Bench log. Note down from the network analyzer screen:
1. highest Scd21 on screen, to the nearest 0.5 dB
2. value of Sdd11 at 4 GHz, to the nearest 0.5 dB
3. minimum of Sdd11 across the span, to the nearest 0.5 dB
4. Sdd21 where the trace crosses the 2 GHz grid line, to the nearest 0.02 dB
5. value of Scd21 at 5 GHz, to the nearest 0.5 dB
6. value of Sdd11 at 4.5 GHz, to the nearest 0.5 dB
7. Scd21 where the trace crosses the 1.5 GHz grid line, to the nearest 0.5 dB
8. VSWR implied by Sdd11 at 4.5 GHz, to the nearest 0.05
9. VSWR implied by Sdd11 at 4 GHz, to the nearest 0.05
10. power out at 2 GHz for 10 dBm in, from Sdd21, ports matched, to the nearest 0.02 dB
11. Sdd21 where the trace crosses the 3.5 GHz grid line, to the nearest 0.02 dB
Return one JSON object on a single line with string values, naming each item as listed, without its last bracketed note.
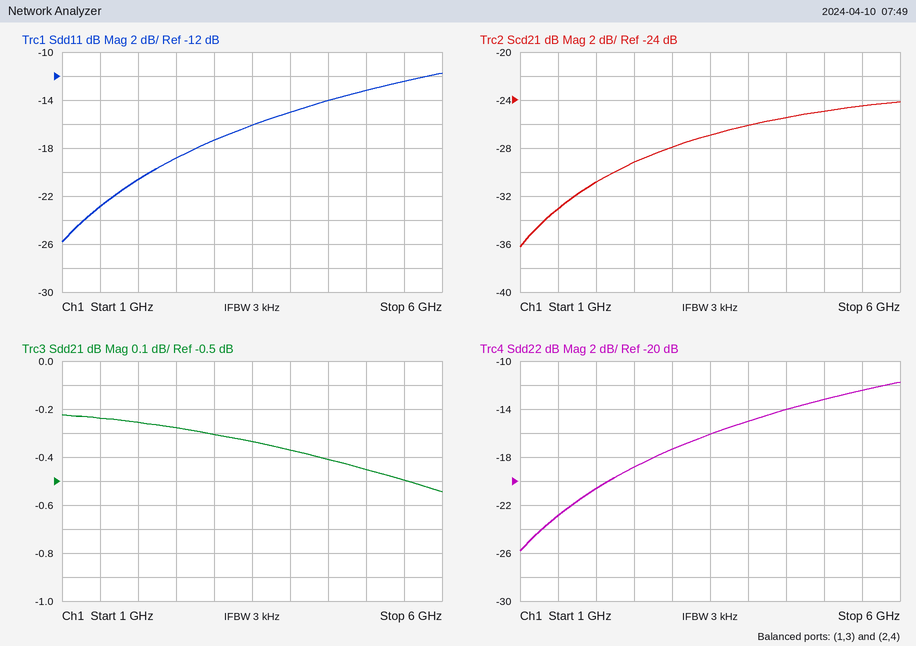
{"highest Scd21 on screen, to the nearest 0.5 dB": "-24.0 dB", "value of Sdd11 at 4 GHz, to the nearest 0.5 dB": "-15.0 dB", "minimum of Sdd11 across the span, to the nearest 0.5 dB": "-26.0 dB", "Sdd21 where the trace crosses the 2 GHz grid line, to the nearest 0.02 dB": "-0.26 dB", "value of Scd21 at 5 GHz, to the nearest 0.5 dB": "-25.0 dB", "value of Sdd11 at 4.5 GHz, to the nearest 0.5 dB": "-14.0 dB", "Scd21 where the trace crosses the 1.5 GHz grid line, to the nearest 0.5 dB": "-33.0 dB", "VSWR implied by Sdd11 at 4.5 GHz, to the nearest 0.05": "1.50", "VSWR implied by Sdd11 at 4 GHz, to the nearest 0.05": "1.45", "power out at 2 GHz for 10 dBm in, from Sdd21, ports matched, to the nearest 0.02 dB": "9.74 dBm", "Sdd21 where the trace crosses the 3.5 GHz grid line, to the nearest 0.02 dB": "-0.34 dB"}
